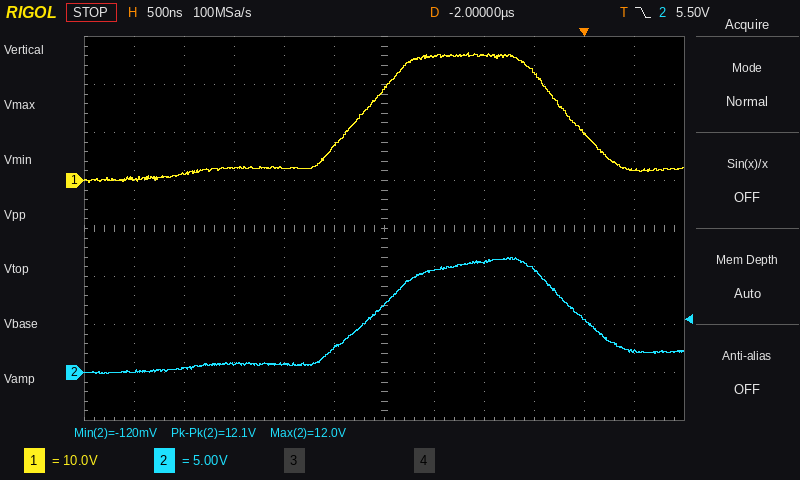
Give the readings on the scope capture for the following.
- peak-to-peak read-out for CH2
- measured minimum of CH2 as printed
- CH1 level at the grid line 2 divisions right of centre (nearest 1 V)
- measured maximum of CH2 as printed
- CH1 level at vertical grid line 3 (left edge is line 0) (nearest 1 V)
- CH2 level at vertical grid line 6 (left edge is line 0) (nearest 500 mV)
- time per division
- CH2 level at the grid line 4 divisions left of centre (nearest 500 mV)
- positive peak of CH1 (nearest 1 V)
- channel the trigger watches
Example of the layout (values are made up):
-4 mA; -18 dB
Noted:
12.1 V; -120 mV; 26 V; 12.0 V; 3 V; 7.0 V; 500 ns; 500 mV; 27 V; CH2
